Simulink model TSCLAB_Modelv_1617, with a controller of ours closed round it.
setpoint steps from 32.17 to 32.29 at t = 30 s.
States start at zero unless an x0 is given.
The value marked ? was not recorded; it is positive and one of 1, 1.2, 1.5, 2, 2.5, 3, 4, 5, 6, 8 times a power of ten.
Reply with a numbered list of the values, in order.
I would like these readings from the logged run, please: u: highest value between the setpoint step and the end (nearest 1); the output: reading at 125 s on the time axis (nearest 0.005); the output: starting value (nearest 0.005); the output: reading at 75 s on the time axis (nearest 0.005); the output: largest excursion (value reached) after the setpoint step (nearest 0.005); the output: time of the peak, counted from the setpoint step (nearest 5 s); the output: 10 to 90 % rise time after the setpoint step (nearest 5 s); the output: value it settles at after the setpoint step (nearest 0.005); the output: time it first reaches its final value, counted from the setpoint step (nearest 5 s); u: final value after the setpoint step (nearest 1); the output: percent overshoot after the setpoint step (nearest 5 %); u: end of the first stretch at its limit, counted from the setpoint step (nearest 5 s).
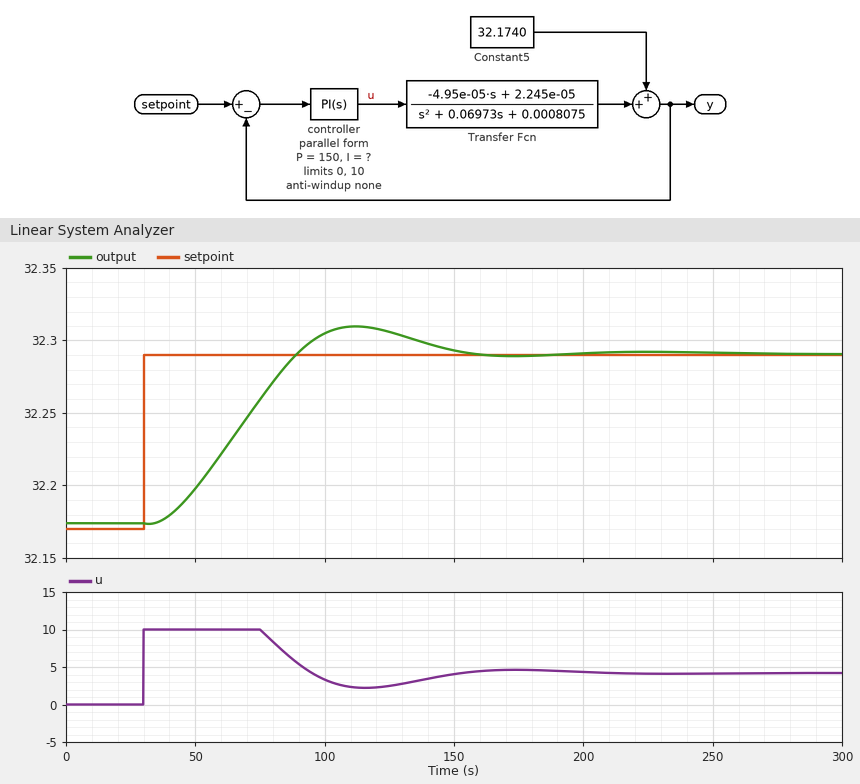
1. 10
2. 32.305
3. 32.175
4. 32.260
5. 32.310
6. 80 s
7. 40 s
8. 32.290
9. 60 s
10. 4
11. 15 %
12. 45 s
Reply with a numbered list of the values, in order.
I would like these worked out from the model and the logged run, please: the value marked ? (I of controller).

1. 1.5
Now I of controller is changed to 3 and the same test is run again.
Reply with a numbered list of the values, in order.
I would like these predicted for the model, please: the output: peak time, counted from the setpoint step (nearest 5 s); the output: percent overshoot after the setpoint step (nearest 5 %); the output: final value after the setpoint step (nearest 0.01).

1. 90 s
2. 40 %
3. 32.29
